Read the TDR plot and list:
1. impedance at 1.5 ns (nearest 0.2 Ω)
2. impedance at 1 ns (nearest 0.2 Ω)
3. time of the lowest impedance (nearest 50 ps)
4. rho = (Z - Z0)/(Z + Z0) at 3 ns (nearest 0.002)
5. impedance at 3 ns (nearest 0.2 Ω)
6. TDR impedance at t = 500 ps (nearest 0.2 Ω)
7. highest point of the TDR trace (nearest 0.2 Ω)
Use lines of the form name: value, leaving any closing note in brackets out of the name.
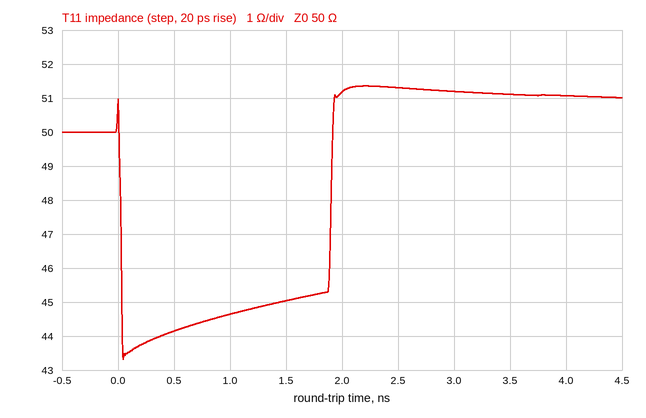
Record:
impedance at 1.5 ns: 45.0 Ω
impedance at 1 ns: 44.6 Ω
time of the lowest impedance: 50 ps
rho = (Z - Z0)/(Z + Z0) at 3 ns: +0.012
impedance at 3 ns: 51.2 Ω
TDR impedance at t = 500 ps: 44.2 Ω
highest point of the TDR trace: 51.4 Ω
